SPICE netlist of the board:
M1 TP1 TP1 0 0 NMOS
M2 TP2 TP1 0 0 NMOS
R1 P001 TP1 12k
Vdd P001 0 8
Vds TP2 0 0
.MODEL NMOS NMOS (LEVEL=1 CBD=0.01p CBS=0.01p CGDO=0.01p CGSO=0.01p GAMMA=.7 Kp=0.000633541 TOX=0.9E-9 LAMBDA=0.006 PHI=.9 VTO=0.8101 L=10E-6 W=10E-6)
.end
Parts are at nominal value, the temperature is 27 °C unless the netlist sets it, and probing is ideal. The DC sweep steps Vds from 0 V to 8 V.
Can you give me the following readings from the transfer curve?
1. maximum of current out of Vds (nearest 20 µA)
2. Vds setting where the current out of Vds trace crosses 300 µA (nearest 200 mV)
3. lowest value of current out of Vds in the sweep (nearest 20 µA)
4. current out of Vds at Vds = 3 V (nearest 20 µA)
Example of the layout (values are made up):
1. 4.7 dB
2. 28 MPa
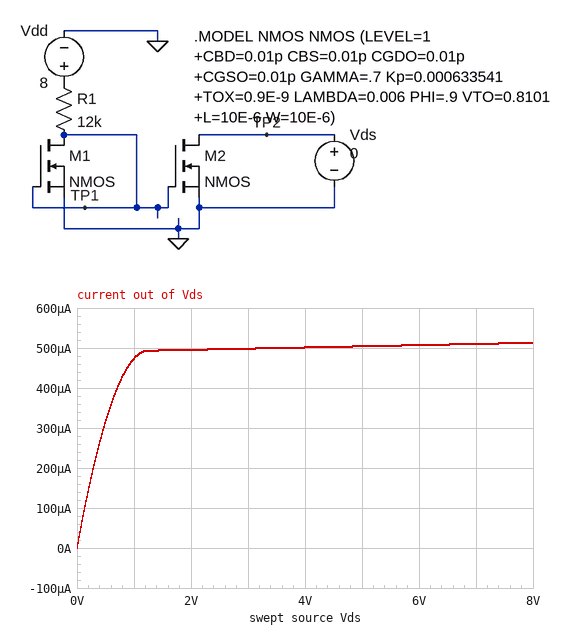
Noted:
1. 520 µA
2. 400 mV
3. 0 A
4. 500 µA
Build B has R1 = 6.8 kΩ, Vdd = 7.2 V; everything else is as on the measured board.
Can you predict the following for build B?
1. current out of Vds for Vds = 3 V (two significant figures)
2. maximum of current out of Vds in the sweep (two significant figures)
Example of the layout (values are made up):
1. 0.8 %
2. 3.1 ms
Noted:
1. 720 µA
2. 740 µA
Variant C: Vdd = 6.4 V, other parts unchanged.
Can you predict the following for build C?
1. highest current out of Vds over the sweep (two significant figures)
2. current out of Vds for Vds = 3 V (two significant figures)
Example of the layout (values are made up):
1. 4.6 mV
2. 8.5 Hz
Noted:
1. 390 µA
2. 380 µA
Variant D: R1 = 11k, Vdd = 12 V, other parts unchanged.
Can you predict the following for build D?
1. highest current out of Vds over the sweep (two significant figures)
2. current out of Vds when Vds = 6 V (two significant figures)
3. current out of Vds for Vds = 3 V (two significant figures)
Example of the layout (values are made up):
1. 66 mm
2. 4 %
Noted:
1. 900 µA
2. 890 µA
3. 870 µA
